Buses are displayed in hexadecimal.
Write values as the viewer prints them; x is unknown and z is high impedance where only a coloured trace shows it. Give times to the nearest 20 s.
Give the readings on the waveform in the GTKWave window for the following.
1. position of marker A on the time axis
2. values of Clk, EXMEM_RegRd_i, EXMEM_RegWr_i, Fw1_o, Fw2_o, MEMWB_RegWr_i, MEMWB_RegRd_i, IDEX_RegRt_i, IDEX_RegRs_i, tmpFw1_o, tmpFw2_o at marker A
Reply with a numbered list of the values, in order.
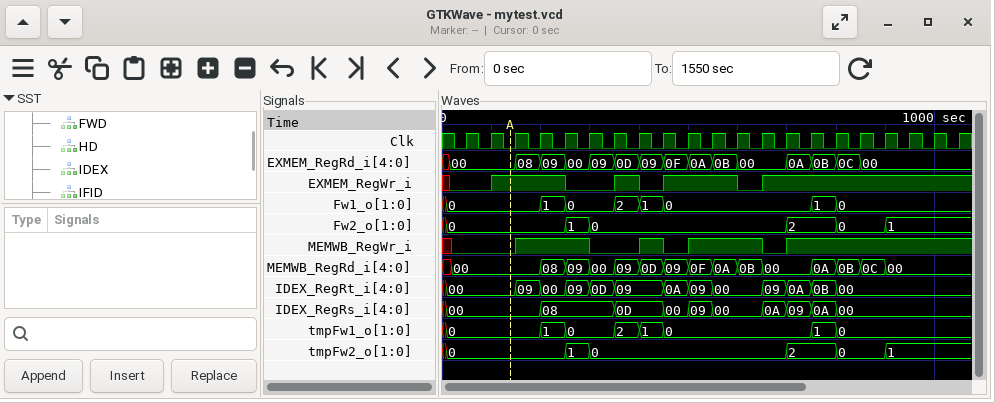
1. 140 s
2. Clk=0, EXMEM_RegRd_i=00, EXMEM_RegWr_i=1, Fw1_o=0, Fw2_o=0, MEMWB_RegWr_i=0, MEMWB_RegRd_i=00, IDEX_RegRt_i=00, IDEX_RegRs_i=00, tmpFw1_o=0, tmpFw2_o=0
